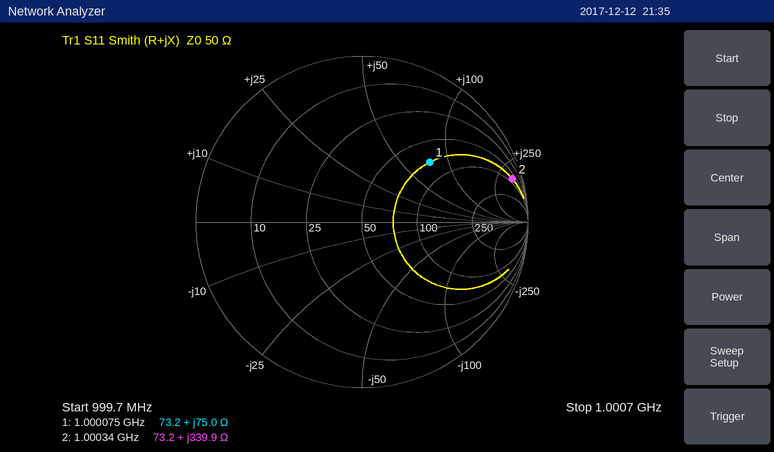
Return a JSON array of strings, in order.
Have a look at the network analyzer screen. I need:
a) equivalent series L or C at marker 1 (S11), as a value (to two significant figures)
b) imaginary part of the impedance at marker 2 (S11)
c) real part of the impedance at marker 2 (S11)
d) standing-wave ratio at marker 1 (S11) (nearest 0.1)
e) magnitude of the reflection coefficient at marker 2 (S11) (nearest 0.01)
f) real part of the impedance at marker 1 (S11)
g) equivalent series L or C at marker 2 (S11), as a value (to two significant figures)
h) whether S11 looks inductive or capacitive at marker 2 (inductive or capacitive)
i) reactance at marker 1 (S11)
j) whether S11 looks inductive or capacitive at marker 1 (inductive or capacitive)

["12 nH", "+339.9 Ω", "73.2 Ω", "3.4", "0.94", "73.2 Ω", "54 nH", "inductive", "+75.0 Ω", "inductive"]
